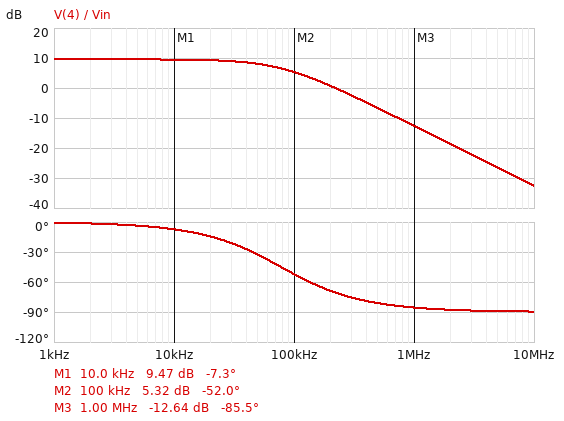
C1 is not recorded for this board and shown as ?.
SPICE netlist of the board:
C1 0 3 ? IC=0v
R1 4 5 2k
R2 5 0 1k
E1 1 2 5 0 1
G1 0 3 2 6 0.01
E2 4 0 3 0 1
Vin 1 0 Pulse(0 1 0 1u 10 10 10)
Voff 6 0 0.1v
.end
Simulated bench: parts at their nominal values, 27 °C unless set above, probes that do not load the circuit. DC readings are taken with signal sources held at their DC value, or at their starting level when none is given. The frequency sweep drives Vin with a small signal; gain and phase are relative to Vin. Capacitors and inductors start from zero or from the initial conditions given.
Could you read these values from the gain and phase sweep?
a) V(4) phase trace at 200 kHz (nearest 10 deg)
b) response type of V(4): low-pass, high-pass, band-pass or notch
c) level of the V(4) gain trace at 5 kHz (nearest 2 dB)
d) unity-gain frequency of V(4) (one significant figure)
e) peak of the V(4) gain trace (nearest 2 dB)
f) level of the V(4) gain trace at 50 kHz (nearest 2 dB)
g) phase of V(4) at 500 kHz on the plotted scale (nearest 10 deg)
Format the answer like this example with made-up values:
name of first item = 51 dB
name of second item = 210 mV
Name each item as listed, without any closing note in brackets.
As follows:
V(4) phase trace at 200 kHz = -70 deg
response type of V(4): low-pass, high-pass, band-pass or notch = low-pass
level of the V(4) gain trace at 5 kHz = 10 dB
unity-gain frequency of V(4) = 200 kHz
peak of the V(4) gain trace = 10 dB
level of the V(4) gain trace at 50 kHz = 8 dB
phase of V(4) at 500 kHz on the plotted scale = -80 deg
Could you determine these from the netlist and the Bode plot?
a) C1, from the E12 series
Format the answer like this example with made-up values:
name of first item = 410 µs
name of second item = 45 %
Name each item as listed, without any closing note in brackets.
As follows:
C1, from the E12 series = 6.8 nF
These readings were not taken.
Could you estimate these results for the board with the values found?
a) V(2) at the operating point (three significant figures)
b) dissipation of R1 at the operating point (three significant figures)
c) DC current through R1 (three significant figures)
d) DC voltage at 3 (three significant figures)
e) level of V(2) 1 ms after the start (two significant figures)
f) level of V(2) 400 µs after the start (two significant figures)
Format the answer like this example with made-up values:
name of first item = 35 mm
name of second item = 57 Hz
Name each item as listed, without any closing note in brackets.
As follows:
V(2) at the operating point = 100 mV
dissipation of R1 at the operating point = 20.0 µW
DC current through R1 = 100 µA
DC voltage at 3 = -300 mV
level of V(2) 1 ms after the start = 100 mV
level of V(2) 400 µs after the start = 100 mV
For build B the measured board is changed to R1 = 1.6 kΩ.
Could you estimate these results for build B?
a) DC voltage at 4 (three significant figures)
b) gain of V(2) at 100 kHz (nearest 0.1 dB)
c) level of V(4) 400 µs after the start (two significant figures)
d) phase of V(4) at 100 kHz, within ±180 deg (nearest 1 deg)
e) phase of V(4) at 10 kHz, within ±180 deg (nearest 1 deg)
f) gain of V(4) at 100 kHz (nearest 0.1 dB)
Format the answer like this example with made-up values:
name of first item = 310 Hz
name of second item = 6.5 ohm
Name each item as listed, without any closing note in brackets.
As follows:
DC voltage at 4 = -260 mV
gain of V(2) at 100 kHz = -2.6 dB
level of V(4) 400 µs after the start = 2.3 V
phase of V(4) at 100 kHz, within ±180 deg = -48 deg
phase of V(4) at 10 kHz, within ±180 deg = -6 deg
gain of V(4) at 100 kHz = 4.8 dB
